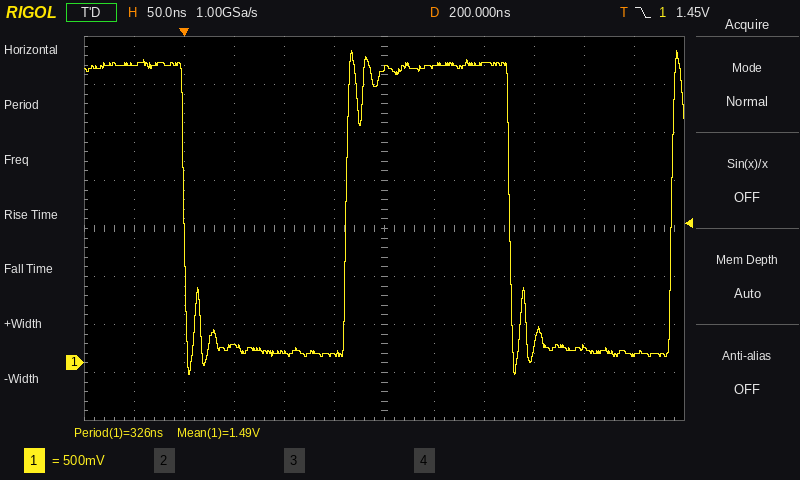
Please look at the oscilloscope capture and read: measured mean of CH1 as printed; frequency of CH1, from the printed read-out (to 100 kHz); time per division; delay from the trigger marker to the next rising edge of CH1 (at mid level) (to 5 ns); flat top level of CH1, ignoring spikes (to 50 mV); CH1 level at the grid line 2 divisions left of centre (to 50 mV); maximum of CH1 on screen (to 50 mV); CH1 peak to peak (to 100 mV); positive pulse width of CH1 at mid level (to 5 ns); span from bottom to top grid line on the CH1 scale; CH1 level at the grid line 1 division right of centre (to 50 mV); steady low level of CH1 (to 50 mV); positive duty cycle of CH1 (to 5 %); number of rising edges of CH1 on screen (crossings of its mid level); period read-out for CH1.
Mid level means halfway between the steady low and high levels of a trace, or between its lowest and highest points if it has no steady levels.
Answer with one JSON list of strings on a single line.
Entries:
["1.49 V", "3.1 MHz", "50 ns", "160 ns", "3.10 V", "100 mV", "3.25 V", "3.40 V", "165 ns", "4 V", "3.10 V", "100 mV", "50 %", "2", "326 ns"]
